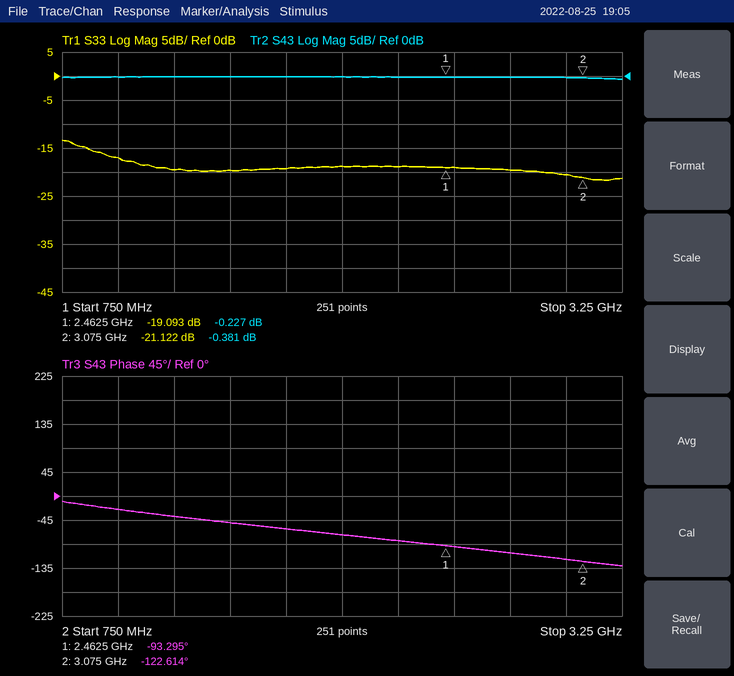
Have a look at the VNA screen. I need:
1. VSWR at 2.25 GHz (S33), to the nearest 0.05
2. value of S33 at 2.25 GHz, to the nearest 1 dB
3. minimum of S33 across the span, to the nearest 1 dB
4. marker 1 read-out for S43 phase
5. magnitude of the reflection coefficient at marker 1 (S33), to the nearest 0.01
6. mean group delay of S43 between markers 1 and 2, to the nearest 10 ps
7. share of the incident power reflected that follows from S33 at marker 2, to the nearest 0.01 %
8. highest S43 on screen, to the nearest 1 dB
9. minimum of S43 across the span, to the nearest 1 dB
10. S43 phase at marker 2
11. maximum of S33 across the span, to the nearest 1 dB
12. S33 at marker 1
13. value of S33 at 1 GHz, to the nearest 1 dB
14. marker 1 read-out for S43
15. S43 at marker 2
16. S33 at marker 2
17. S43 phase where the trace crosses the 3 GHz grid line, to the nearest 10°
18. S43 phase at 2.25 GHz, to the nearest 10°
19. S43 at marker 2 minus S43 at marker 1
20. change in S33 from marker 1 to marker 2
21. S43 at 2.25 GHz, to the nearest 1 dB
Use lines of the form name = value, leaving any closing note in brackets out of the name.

VSWR at 2.25 GHz (S33), to the nearest 0.05 = 1.25
value of S33 at 2.25 GHz, to the nearest 1 dB = -19 dB
minimum of S33 across the span, to the nearest 1 dB = -22 dB
marker 1 read-out for S43 phase = -93.295°
magnitude of the reflection coefficient at marker 1 (S33), to the nearest 0.01 = 0.11
mean group delay of S43 between markers 1 and 2, to the nearest 10 ps = 130 ps
share of the incident power reflected that follows from S33 at marker 2, to the nearest 0.01 % = 0.77 %
highest S43 on screen, to the nearest 1 dB = 0 dB
minimum of S43 across the span, to the nearest 1 dB = -1 dB
S43 phase at marker 2 = -122.614°
maximum of S33 across the span, to the nearest 1 dB = -13 dB
S33 at marker 1 = -19.093 dB
value of S33 at 1 GHz, to the nearest 1 dB = -17 dB
marker 1 read-out for S43 = -0.227 dB
S43 at marker 2 = -0.381 dB
S33 at marker 2 = -21.122 dB
S43 phase where the trace crosses the 3 GHz grid line, to the nearest 10° = -120°
S43 phase at 2.25 GHz, to the nearest 10° = -80°
S43 at marker 2 minus S43 at marker 1 = -0.154 dB
change in S33 from marker 1 to marker 2 = -2.029 dB
S43 at 2.25 GHz, to the nearest 1 dB = 0 dB
